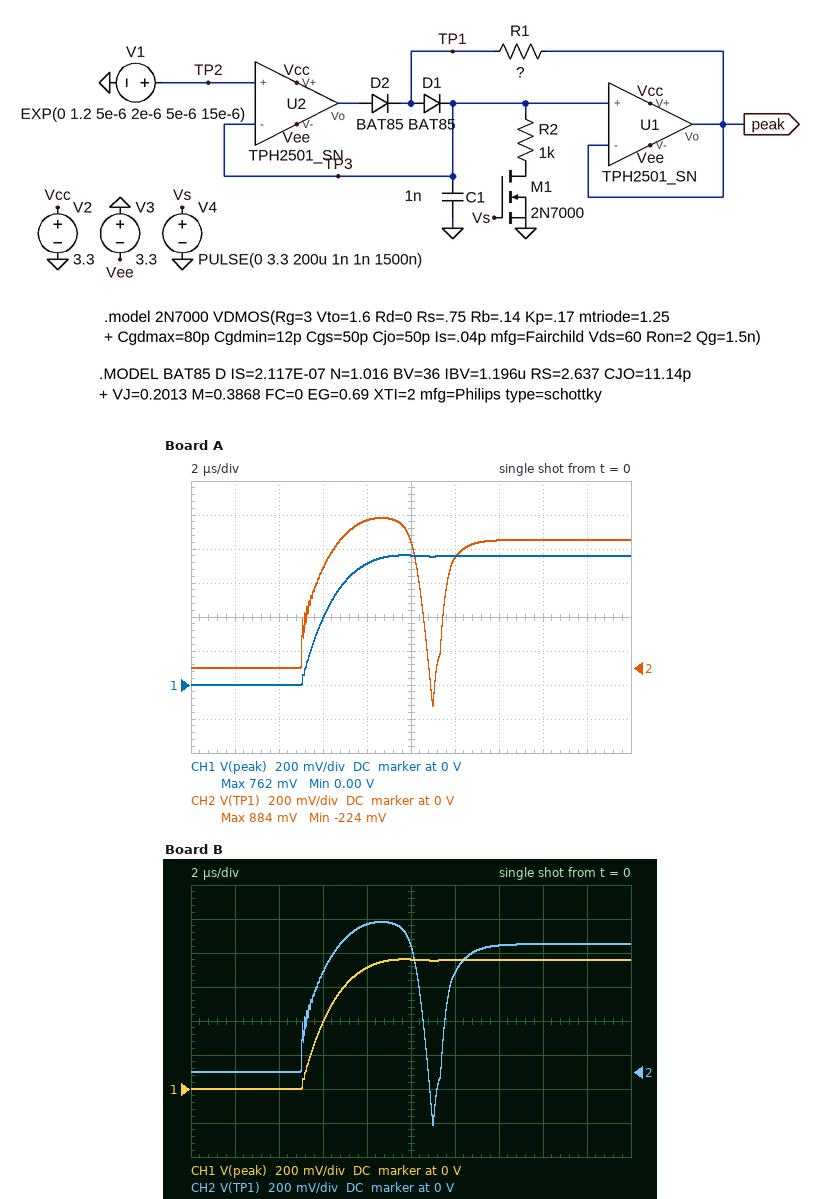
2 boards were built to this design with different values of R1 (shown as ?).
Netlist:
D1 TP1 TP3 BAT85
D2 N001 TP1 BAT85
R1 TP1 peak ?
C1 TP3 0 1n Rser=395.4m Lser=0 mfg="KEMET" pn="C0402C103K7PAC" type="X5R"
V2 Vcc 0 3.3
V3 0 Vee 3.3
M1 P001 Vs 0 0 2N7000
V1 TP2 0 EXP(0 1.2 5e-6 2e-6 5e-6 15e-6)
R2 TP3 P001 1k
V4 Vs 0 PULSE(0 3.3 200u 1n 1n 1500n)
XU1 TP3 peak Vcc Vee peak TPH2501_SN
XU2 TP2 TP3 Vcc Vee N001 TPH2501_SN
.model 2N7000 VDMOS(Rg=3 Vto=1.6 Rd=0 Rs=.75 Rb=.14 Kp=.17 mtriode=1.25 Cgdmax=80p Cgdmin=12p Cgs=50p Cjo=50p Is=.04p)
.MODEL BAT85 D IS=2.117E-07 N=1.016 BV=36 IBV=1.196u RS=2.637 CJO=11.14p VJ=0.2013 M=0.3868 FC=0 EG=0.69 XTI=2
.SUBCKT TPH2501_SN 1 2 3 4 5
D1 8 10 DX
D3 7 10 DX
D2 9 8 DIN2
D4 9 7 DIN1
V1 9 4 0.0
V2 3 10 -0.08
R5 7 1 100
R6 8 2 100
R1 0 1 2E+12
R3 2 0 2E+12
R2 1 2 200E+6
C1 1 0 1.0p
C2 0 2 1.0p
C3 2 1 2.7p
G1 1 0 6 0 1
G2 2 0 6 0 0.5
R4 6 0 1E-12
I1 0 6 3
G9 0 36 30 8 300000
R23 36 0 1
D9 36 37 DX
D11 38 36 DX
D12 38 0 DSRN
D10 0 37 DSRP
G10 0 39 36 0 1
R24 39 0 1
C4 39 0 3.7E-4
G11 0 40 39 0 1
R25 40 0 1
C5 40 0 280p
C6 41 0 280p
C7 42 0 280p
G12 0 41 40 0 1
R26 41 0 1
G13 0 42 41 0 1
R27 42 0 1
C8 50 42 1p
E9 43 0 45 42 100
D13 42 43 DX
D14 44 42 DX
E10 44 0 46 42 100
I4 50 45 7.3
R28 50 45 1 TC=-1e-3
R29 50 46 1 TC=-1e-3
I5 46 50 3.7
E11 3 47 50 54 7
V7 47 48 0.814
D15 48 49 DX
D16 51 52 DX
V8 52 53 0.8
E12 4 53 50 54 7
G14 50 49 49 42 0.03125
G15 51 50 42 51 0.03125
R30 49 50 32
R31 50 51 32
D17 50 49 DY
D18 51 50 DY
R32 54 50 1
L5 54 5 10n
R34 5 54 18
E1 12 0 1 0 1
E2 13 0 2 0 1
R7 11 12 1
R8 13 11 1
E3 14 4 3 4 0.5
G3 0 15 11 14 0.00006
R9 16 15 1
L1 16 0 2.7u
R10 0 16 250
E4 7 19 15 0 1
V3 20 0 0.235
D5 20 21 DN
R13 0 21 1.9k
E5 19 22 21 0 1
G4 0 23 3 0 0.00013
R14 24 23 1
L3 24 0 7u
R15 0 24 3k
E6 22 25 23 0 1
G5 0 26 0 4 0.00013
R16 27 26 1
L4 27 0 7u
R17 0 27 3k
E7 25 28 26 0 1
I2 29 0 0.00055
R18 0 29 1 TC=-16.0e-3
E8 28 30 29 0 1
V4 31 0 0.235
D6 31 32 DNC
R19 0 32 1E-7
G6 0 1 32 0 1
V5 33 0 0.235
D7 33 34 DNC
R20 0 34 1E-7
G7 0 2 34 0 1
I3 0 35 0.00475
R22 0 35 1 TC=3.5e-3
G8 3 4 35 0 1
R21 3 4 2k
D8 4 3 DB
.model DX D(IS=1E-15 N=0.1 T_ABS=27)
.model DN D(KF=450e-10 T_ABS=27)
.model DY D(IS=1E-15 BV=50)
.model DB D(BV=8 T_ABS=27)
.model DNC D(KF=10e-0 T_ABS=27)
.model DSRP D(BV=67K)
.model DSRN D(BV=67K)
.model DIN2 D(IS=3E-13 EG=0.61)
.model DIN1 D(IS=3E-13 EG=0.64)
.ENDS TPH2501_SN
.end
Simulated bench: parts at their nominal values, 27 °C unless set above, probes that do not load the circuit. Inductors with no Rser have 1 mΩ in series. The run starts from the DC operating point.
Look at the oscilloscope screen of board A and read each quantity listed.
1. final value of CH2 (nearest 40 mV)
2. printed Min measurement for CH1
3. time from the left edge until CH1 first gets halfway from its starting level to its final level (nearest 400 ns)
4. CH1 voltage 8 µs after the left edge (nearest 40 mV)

760 mV
0.00 V
6.0 µs
720 mV
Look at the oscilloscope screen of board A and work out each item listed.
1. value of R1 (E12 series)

47 kΩ
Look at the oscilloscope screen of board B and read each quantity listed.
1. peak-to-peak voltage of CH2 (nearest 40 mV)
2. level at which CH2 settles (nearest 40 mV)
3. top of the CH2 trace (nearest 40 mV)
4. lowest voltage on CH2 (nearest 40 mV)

1.20 V
760 mV
880 mV
-320 mV
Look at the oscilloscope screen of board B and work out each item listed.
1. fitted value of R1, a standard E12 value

56 kΩ
